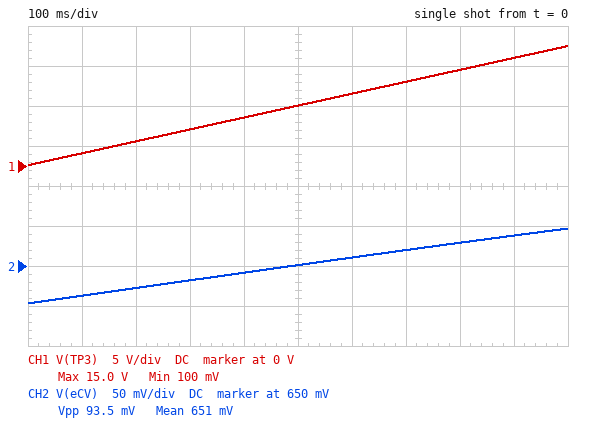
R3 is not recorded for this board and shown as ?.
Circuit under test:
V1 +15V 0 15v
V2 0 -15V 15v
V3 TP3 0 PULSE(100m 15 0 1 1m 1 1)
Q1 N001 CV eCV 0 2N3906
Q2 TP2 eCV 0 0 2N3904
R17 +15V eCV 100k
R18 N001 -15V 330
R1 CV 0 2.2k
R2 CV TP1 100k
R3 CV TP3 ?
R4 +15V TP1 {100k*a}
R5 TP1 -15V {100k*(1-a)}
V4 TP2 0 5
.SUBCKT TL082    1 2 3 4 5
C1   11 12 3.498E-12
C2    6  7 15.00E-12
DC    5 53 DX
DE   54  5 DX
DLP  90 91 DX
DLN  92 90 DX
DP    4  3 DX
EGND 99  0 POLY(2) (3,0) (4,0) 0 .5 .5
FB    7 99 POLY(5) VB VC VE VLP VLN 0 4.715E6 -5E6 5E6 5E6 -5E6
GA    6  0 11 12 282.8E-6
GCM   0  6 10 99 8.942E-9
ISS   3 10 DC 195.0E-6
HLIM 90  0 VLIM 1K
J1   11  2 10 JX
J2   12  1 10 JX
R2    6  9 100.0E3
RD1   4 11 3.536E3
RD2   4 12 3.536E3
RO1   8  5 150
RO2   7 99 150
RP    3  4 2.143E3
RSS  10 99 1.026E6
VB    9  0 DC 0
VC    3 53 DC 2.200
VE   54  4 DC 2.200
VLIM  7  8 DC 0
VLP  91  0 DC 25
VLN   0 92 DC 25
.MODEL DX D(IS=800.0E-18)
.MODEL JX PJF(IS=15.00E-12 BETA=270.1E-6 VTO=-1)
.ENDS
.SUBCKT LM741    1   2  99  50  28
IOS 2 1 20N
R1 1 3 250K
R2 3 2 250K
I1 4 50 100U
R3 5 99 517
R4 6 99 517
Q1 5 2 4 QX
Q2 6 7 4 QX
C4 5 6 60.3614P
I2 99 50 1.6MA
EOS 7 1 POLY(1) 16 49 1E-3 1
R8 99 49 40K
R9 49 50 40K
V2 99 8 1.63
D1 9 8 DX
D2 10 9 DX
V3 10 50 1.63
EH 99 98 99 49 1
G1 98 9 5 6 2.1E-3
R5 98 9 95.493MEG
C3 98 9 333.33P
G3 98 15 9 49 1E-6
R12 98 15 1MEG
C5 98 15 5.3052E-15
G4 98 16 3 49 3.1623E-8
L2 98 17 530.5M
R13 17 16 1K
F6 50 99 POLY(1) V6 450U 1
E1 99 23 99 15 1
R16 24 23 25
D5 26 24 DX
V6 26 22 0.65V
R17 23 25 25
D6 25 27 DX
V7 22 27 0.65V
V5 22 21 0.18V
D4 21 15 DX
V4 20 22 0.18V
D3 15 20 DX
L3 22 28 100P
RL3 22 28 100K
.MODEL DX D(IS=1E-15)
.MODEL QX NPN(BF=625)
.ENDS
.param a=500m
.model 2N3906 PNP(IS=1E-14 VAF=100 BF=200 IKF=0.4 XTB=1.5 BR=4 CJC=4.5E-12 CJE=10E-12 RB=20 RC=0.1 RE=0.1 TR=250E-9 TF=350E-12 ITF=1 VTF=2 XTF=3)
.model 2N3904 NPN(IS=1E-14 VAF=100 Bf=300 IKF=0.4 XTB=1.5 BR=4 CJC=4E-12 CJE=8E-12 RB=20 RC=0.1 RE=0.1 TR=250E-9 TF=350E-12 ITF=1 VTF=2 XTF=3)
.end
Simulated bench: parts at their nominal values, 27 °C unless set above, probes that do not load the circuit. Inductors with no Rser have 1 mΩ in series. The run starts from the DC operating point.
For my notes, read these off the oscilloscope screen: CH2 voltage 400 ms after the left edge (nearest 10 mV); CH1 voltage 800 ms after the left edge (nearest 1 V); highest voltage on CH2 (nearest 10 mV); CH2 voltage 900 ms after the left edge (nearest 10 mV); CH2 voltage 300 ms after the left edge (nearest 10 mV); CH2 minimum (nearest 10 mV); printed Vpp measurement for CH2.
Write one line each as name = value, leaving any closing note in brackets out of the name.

CH2 voltage 400 ms after the left edge = 640 mV
CH1 voltage 800 ms after the left edge = 12 V
highest voltage on CH2 = 700 mV
CH2 voltage 900 ms after the left edge = 690 mV
CH2 voltage 300 ms after the left edge = 630 mV
CH2 minimum = 600 mV
printed Vpp measurement for CH2 = 93.5 mV
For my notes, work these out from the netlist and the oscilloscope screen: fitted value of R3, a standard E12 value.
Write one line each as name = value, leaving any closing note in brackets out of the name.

fitted value of R3, a standard E12 value = 330 kΩ
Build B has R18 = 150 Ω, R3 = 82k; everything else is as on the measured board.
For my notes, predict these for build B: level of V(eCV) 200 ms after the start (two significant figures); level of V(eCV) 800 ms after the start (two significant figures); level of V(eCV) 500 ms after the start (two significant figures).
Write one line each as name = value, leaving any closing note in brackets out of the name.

level of V(eCV) 200 ms after the start = 680 mV
level of V(eCV) 800 ms after the start = 760 mV
level of V(eCV) 500 ms after the start = 750 mV
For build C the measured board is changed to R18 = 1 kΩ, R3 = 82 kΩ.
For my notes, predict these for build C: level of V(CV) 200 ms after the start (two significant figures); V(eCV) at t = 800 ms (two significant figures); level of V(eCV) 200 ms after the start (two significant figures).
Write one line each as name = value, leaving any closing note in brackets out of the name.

level of V(CV) 200 ms after the start = 80 mV
V(eCV) at t = 800 ms = 760 mV
level of V(eCV) 200 ms after the start = 680 mV
